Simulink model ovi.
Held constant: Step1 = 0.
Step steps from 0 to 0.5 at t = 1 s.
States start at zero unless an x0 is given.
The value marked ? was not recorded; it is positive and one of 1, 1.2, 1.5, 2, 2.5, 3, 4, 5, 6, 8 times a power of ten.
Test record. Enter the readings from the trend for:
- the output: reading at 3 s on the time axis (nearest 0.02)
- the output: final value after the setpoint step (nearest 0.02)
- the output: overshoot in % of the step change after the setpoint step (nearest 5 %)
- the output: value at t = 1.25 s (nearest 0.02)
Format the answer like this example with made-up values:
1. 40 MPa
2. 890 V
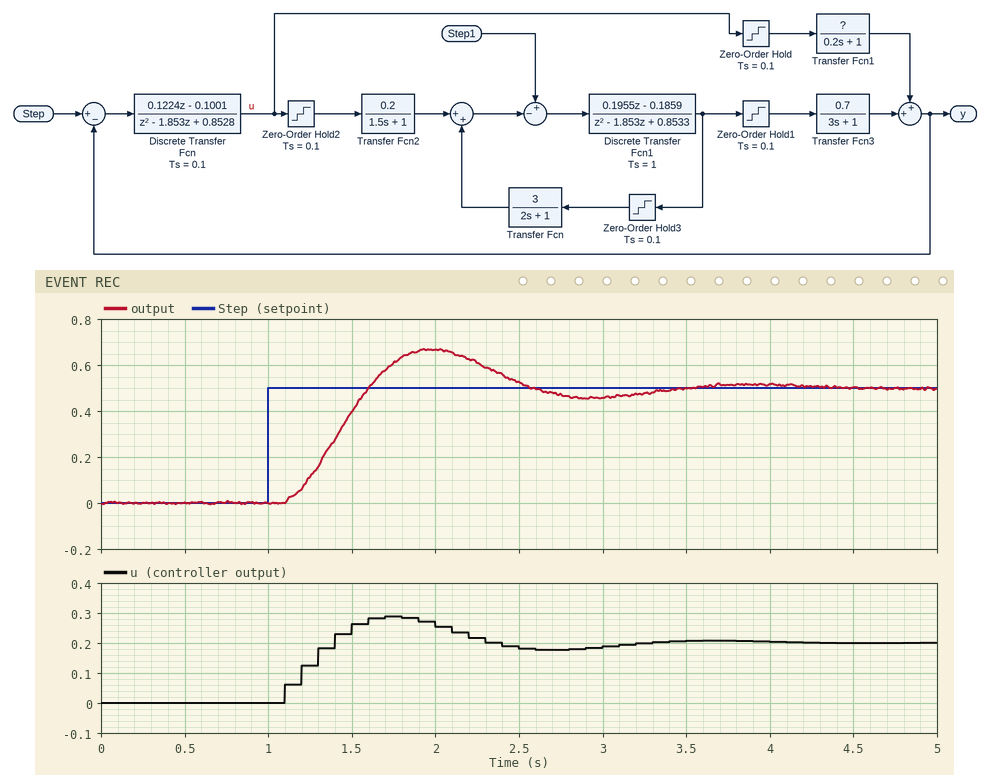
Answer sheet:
1. 0.46
2. 0.50
3. 35 %
4. 0.12
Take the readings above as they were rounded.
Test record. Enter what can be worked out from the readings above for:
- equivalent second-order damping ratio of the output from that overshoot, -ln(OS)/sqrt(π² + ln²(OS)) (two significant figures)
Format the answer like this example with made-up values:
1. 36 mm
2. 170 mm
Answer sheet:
1. 0.32
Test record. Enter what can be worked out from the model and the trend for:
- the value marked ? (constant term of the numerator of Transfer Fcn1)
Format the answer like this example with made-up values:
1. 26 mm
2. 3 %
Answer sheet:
1. 2.5
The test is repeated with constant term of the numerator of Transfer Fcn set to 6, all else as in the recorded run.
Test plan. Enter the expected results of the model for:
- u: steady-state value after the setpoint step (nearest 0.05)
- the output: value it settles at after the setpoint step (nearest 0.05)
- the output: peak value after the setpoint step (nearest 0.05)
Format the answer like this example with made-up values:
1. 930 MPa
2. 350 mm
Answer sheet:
1. 0.20
2. 0.50
3. 0.65
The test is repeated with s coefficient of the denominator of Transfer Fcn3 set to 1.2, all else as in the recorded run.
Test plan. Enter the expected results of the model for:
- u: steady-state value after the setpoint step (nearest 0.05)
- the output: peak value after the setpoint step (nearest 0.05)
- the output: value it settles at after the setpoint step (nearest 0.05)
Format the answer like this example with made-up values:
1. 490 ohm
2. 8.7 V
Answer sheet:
1. 0.20
2. 0.65
3. 0.50
